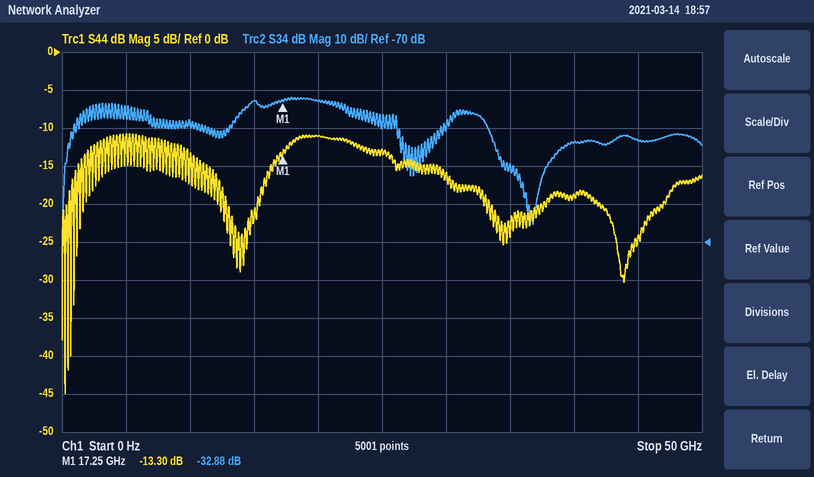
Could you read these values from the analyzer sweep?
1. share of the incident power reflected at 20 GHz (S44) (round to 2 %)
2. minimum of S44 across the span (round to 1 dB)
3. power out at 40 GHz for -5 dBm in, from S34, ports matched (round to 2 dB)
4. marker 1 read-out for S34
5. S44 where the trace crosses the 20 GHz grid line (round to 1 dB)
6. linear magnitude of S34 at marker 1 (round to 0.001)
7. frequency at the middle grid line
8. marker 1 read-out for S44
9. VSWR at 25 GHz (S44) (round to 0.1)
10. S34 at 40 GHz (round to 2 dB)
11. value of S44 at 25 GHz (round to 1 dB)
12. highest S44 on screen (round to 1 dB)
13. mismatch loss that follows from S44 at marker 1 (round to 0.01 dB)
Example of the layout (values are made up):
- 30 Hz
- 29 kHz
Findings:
- 8 %
- -45 dB
- -48 dBm
- -32.88 dB
- -11 dB
- 0.023
- 25 GHz
- -13.30 dB
- 1.6
- -44 dB
- -13 dB
- -11 dB
- 0.21 dB
